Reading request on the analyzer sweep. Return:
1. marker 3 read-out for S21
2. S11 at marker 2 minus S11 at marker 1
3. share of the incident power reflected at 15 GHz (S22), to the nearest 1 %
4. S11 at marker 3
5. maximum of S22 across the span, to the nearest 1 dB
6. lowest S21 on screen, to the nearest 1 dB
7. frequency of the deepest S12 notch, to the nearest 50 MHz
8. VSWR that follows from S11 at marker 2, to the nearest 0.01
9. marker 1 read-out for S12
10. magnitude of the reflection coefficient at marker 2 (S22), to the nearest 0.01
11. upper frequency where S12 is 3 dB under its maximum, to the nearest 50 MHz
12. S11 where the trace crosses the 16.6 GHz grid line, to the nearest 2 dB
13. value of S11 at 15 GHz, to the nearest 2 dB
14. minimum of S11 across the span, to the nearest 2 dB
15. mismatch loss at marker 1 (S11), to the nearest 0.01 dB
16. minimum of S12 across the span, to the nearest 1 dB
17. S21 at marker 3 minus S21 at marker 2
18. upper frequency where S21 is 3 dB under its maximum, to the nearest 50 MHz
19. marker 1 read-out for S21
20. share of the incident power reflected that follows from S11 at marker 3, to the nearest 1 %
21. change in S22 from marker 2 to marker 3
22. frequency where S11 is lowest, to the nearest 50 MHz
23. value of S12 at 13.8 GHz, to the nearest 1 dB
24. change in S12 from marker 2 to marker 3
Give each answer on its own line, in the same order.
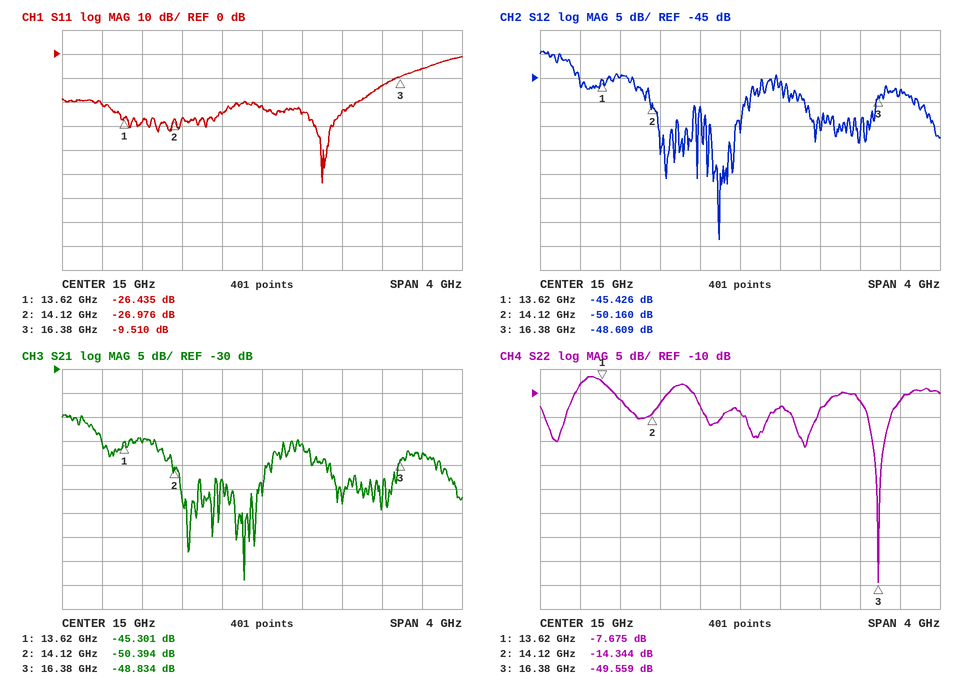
-48.834 dB
-0.541 dB
4 %
-9.510 dB
-7 dB
-74 dB
14.80 GHz
1.09
-45.426 dB
0.19
13.30 GHz
-6 dB
-22 dB
-54 dB
0.01 dB
-79 dB
1.560 dB
13.30 GHz
-45.301 dB
11 %
-35.215 dB
15.60 GHz
-45 dB
1.551 dB
